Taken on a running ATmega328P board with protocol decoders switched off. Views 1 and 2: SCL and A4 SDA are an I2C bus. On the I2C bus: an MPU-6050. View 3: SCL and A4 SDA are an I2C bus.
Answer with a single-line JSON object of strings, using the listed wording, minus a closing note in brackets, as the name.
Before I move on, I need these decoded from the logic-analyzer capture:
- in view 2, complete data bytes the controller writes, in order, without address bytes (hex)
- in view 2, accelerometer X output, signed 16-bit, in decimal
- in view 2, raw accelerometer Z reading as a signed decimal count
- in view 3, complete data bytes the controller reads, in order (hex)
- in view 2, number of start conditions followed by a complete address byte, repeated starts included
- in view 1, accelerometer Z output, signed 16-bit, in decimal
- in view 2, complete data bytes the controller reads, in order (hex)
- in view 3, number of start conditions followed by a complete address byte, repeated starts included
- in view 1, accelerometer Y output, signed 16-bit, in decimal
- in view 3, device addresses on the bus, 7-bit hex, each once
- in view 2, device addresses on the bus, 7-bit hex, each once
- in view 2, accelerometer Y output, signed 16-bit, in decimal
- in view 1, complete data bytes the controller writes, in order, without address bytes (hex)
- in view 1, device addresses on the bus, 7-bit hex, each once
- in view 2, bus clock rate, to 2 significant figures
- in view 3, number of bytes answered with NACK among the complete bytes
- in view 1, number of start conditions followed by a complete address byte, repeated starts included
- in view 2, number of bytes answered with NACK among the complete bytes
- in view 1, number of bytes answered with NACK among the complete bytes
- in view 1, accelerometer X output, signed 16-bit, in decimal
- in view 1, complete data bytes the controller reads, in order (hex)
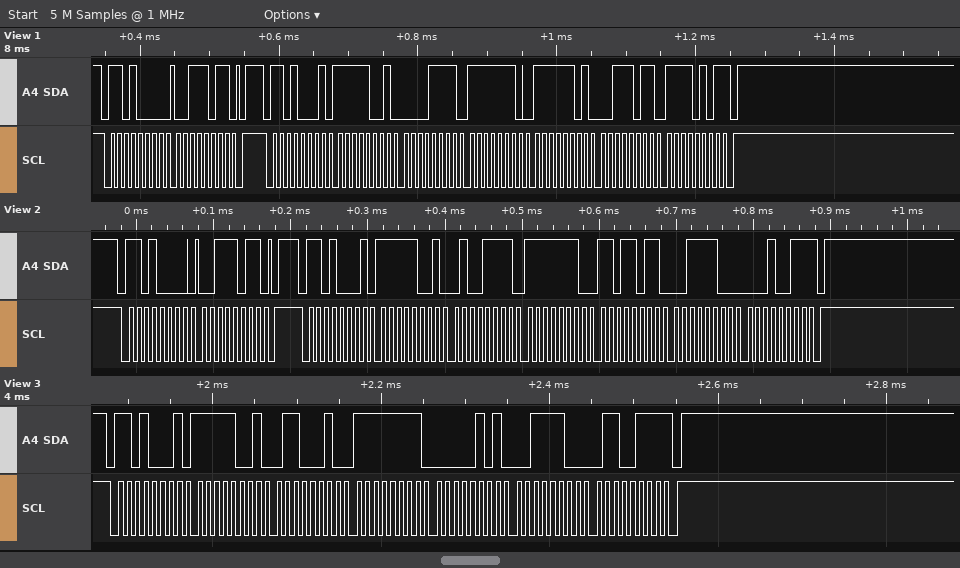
{"in view 2, complete data bytes the controller writes, in order, without address bytes": "3B", "in view 2, accelerometer X output, signed 16-bit, in decimal": "-1713", "in view 2, raw accelerometer Z reading as a signed decimal count": "15379", "in view 3, complete data bytes the controller reads, in order": "F9 62 FF 05 3C 67", "in view 2, number of start conditions followed by a complete address byte, repeated starts included": "2", "in view 1, accelerometer Z output, signed 16-bit, in decimal": "15349", "in view 2, complete data bytes the controller reads, in order": "F9 4F FE DB 3C 13", "in view 3, number of start conditions followed by a complete address byte, repeated starts included": "1", "in view 1, accelerometer Y output, signed 16-bit, in decimal": "-259", "in view 3, device addresses on the bus, 7-bit hex, each once": "0x68", "in view 2, device addresses on the bus, 7-bit hex, each once": "0x68", "in view 2, accelerometer Y output, signed 16-bit, in decimal": "-293", "in view 1, complete data bytes the controller writes, in order, without address bytes": "3B", "in view 1, device addresses on the bus, 7-bit hex, each once": "0x68", "in view 2, bus clock rate, to 2 significant figures": "100 kHz", "in view 3, number of bytes answered with NACK among the complete bytes": "1", "in view 1, number of start conditions followed by a complete address byte, repeated starts included": "2", "in view 2, number of bytes answered with NACK among the complete bytes": "1", "in view 1, number of bytes answered with NACK among the complete bytes": "1", "in view 1, accelerometer X output, signed 16-bit, in decimal": "-1777", "in view 1, complete data bytes the controller reads, in order": "F9 0F FE FD 3B F5"}
